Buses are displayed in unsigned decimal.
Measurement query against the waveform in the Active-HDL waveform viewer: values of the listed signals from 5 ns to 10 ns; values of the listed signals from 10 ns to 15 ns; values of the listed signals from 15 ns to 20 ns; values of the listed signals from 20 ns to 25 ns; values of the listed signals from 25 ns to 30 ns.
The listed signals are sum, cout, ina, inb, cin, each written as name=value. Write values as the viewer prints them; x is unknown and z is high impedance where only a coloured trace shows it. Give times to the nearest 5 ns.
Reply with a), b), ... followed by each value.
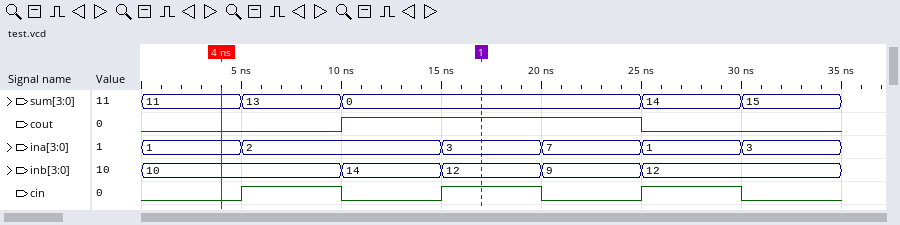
a) sum=13, cout=0, ina=2, inb=10, cin=1
b) sum=0, cout=1, ina=2, inb=14, cin=0
c) sum=0, cout=1, ina=3, inb=12, cin=1
d) sum=0, cout=1, ina=7, inb=9, cin=0
e) sum=14, cout=0, ina=1, inb=12, cin=1
